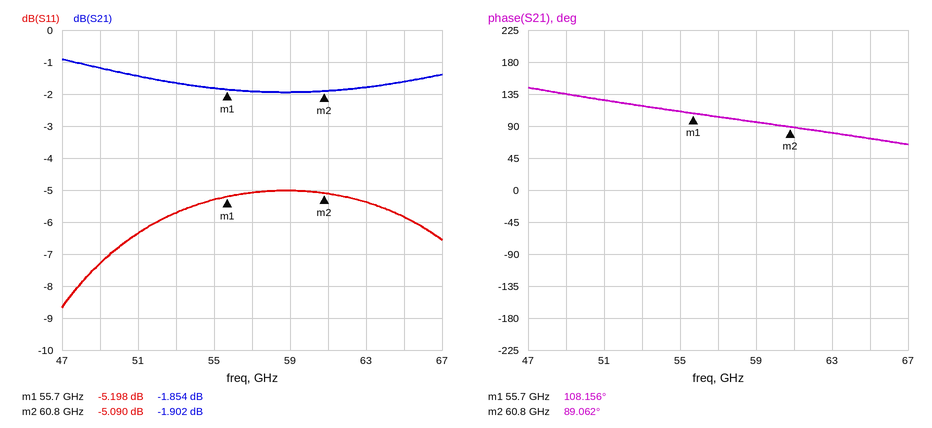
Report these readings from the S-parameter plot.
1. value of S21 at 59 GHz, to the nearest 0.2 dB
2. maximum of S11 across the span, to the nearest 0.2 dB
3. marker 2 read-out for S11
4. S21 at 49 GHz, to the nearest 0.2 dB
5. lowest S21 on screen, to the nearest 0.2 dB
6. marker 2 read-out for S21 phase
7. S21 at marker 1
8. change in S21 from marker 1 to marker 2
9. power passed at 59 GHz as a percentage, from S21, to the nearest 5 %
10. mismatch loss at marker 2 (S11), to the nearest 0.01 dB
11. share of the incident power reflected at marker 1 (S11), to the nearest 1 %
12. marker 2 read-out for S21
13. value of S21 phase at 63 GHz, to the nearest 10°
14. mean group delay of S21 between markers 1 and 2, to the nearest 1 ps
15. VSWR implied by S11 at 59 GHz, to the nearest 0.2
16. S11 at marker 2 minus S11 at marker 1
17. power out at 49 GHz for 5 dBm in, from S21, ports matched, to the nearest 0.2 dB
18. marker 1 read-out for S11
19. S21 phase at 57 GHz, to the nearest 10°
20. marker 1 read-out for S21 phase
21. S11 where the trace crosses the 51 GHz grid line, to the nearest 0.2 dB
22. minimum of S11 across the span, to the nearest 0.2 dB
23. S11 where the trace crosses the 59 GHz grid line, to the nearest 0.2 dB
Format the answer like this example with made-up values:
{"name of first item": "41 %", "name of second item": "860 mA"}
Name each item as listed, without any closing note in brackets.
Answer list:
{"value of S21 at 59 GHz, to the nearest 0.2 dB": "-2.0 dB", "maximum of S11 across the span, to the nearest 0.2 dB": "-5.0 dB", "marker 2 read-out for S11": "-5.090 dB", "S21 at 49 GHz, to the nearest 0.2 dB": "-1.2 dB", "lowest S21 on screen, to the nearest 0.2 dB": "-2.0 dB", "marker 2 read-out for S21 phase": "89.062°", "S21 at marker 1": "-1.854 dB", "change in S21 from marker 1 to marker 2": "-0.048 dB", "power passed at 59 GHz as a percentage, from S21, to the nearest 5 %": "65 %", "mismatch loss at marker 2 (S11), to the nearest 0.01 dB": "1.61 dB", "share of the incident power reflected at marker 1 (S11), to the nearest 1 %": "30 %", "marker 2 read-out for S21": "-1.902 dB", "value of S21 phase at 63 GHz, to the nearest 10°": "80°", "mean group delay of S21 between markers 1 and 2, to the nearest 1 ps": "10 ps", "VSWR implied by S11 at 59 GHz, to the nearest 0.2": "3.6", "S11 at marker 2 minus S11 at marker 1": "0.108 dB", "power out at 49 GHz for 5 dBm in, from S21, ports matched, to the nearest 0.2 dB": "3.8 dBm", "marker 1 read-out for S11": "-5.198 dB", "S21 phase at 57 GHz, to the nearest 10°": "100°", "marker 1 read-out for S21 phase": "108.156°", "S11 where the trace crosses the 51 GHz grid line, to the nearest 0.2 dB": "-6.4 dB", "minimum of S11 across the span, to the nearest 0.2 dB": "-8.6 dB", "S11 where the trace crosses the 59 GHz grid line, to the nearest 0.2 dB": "-5.0 dB"}
